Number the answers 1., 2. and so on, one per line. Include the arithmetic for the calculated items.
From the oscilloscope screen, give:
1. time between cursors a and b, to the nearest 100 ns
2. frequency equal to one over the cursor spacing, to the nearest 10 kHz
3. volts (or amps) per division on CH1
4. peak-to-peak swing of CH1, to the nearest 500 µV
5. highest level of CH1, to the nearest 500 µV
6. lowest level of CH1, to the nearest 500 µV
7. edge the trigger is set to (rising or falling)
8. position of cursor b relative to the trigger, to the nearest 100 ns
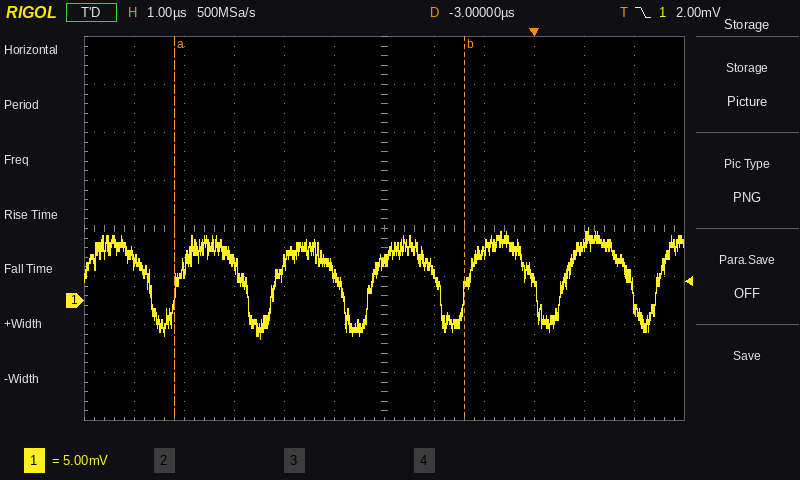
1. 5.8 µs
2. 1 / 5.8 µs ≈ 170 kHz
3. 5 mV
4. 7.5 mV − (-4.0 mV) = 11.5 mV
5. 7.5 mV
6. -4.0 mV
7. falling
8. -1.4 µs
